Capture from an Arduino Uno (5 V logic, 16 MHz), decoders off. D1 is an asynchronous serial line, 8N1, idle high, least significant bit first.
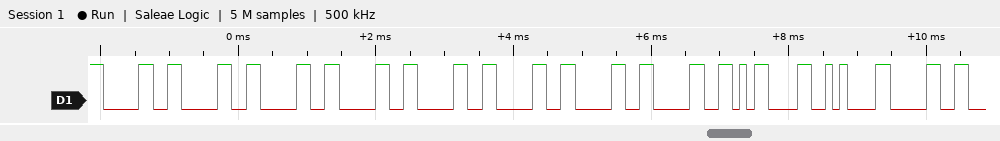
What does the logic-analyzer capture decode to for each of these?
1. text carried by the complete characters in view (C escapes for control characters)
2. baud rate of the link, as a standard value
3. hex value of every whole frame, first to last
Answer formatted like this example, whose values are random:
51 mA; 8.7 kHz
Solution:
"00000000\r\n0"; 9600 baud; 0x30 0x30 0x30 0x30 0x30 0x30 0x30 0x30 0x0D 0x0A 0x30
